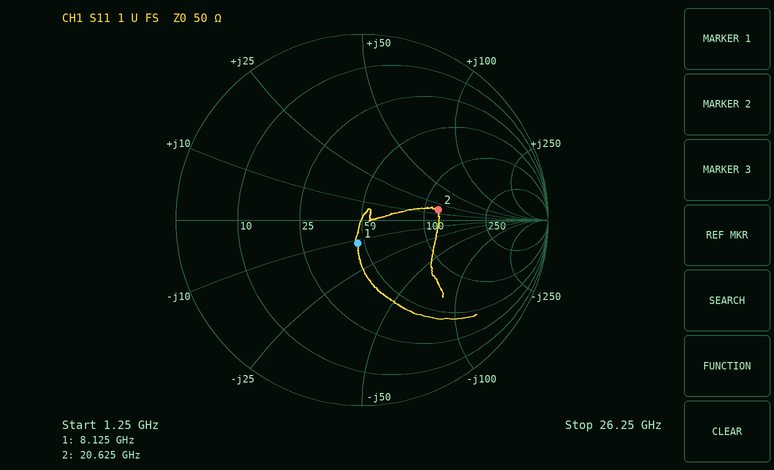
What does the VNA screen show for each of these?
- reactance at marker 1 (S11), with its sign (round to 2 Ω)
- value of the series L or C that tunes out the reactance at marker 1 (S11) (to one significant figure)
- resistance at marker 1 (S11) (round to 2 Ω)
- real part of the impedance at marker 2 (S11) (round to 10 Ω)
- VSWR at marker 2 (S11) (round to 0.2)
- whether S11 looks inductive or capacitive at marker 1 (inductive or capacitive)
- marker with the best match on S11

-12 Ω
200 pH
46 Ω
120 Ω
2.4
capacitive
marker 1
